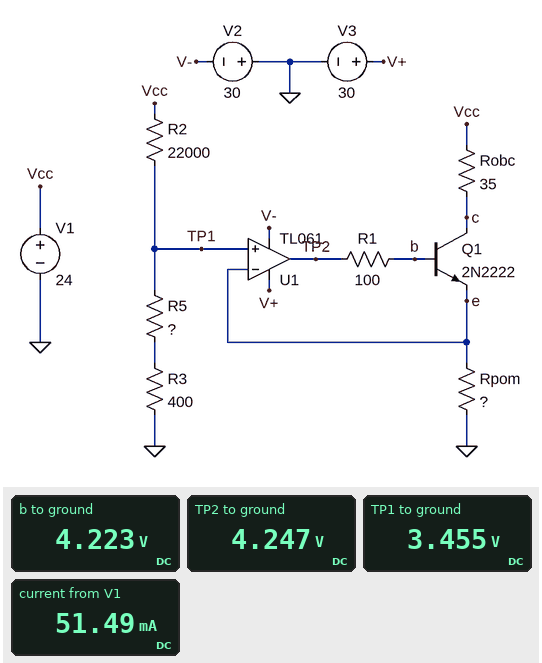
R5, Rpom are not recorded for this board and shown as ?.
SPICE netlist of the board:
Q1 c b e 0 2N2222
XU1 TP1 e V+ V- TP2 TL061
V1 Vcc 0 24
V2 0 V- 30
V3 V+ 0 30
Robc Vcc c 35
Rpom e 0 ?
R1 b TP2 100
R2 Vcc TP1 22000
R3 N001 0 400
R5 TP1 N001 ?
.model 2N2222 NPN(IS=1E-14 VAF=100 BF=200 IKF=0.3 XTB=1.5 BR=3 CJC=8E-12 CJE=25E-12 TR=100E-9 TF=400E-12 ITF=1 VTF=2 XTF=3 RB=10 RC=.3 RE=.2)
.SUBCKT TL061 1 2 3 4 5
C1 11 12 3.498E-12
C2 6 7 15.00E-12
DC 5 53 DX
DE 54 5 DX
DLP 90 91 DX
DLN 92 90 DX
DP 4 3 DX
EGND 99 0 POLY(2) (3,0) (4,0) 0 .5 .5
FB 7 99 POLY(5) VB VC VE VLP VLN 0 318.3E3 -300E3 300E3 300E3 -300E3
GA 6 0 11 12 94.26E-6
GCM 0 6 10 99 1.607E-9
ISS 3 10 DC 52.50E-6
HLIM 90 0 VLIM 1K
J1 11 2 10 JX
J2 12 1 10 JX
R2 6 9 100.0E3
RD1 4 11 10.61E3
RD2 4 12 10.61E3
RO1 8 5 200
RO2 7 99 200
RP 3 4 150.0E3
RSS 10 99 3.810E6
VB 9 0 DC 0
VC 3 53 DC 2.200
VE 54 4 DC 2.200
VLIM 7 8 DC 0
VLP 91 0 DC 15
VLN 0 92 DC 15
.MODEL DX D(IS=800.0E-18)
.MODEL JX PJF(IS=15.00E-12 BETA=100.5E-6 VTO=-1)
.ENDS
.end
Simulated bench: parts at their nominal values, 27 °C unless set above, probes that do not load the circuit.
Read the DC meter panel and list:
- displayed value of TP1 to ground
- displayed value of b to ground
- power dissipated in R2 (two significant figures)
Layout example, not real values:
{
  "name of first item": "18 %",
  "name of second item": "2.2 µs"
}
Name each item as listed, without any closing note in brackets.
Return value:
{
  "displayed value of TP1 to ground": "3.455 V",
  "displayed value of b to ground": "4.223 V",
  "power dissipated in R2": "19 mW"
}
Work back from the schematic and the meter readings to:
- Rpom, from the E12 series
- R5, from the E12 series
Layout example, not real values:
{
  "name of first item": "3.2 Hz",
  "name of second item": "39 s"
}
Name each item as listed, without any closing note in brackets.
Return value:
{
  "Rpom, from the E12 series": "68 Ω",
  "R5, from the E12 series": "3.3 kΩ"
}
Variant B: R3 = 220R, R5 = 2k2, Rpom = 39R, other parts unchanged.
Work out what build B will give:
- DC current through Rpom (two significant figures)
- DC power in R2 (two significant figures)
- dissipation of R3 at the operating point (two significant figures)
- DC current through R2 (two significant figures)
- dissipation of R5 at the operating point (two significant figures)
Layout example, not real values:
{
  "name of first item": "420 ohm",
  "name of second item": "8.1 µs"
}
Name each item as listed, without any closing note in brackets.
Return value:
{
  "DC current through Rpom": "61 mA",
  "DC power in R2": "21 mW",
  "dissipation of R3 at the operating point": "210 µW",
  "DC current through R2": "980 µA",
  "dissipation of R5 at the operating point": "2.1 mW"
}
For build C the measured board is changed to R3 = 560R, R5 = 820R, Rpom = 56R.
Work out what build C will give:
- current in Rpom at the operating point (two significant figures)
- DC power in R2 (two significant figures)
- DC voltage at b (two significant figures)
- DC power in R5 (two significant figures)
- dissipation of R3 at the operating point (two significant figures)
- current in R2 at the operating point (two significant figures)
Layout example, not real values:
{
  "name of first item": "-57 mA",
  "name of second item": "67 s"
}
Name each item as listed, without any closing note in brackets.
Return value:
{
  "current in Rpom at the operating point": "25 mA",
  "DC power in R2": "23 mW",
  "DC voltage at b": "2.2 V",
  "DC power in R5": "860 µW",
  "dissipation of R3 at the operating point": "590 µW",
  "current in R2 at the operating point": "1.0 mA"
}
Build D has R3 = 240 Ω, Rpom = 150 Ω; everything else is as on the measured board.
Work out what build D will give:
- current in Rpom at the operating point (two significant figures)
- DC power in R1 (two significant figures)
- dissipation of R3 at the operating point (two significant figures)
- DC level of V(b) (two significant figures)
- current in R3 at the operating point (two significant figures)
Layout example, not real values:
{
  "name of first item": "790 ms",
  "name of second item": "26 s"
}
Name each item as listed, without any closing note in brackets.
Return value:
{
  "current in Rpom at the operating point": "22 mA",
  "DC power in R1": "970 nW",
  "dissipation of R3 at the operating point": "210 µW",
  "DC level of V(b)": "4.1 V",
  "current in R3 at the operating point": "940 µA"
}
